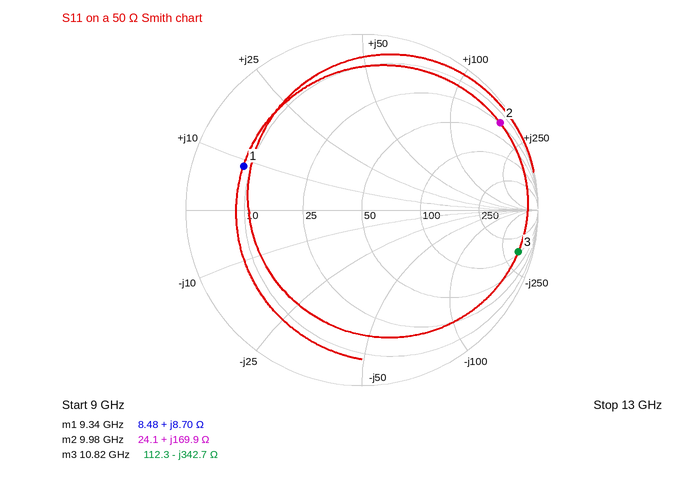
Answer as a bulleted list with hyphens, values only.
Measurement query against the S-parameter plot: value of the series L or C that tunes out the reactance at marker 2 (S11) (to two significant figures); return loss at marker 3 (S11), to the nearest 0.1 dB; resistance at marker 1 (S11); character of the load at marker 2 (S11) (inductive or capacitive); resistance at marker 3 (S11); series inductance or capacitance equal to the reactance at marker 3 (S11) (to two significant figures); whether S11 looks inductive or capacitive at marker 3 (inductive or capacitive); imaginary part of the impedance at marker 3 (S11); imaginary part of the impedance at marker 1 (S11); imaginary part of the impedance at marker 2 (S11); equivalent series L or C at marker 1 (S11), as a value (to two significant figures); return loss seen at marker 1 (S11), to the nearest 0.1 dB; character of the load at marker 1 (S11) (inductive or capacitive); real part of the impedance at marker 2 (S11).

- 94 fF
- 0.7 dB
- 8.48 Ω
- inductive
- 112.3 Ω
- 43 fF
- capacitive
- -342.7 Ω
- +8.70 Ω
- +169.9 Ω
- 150 pH
- 2.9 dB
- inductive
- 24.1 Ω
